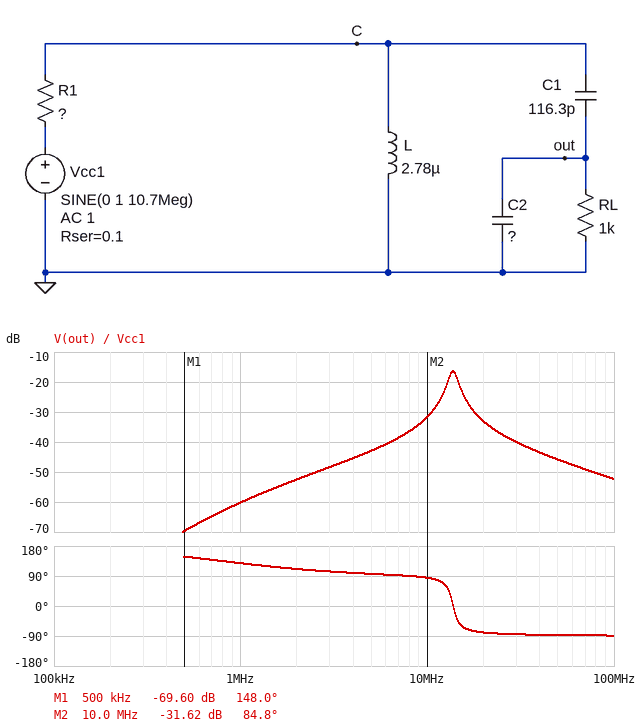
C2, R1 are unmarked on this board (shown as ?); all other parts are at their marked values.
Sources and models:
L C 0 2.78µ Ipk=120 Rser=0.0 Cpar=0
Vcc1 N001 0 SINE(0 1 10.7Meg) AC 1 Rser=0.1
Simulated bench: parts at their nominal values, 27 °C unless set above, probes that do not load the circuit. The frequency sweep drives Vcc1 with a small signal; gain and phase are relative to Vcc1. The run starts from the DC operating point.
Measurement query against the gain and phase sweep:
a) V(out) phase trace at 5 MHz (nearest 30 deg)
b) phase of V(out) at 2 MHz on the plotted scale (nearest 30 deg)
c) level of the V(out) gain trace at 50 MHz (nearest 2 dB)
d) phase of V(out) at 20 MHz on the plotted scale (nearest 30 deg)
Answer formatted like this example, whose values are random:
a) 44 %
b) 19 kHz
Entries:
a) 90 deg
b) 120 deg
c) -46 dB
d) -90 deg
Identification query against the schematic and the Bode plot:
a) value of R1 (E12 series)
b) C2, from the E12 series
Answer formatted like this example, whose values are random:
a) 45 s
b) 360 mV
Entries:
a) 8.2 kΩ
b) 82 pF
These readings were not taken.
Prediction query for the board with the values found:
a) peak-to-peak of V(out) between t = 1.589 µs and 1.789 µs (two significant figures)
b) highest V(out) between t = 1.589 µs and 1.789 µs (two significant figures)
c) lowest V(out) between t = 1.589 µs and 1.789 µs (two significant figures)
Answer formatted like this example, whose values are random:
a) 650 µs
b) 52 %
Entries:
a) 67 mV
b) 33 mV
c) -33 mV
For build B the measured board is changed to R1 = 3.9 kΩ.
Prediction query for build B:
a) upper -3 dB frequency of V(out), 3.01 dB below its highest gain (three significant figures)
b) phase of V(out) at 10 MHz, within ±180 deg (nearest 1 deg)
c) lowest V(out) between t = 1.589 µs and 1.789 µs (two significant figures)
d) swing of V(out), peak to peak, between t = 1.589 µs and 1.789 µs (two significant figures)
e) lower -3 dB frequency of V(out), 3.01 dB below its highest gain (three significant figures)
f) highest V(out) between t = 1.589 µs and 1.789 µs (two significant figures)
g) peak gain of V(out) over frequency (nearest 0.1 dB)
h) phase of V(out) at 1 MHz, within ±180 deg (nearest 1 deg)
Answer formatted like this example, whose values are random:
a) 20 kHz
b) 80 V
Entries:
a) 14.8 MHz
b) 82 deg
c) -69 mV
d) 140 mV
e) 12.8 MHz
f) 69 mV
g) -12.0 dB
h) 128 deg
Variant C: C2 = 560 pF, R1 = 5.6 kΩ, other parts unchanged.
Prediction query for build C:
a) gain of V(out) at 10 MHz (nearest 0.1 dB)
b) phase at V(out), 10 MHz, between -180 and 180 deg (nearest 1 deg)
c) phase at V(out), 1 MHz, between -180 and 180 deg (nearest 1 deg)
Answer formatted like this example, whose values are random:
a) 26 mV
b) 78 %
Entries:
a) -22.0 dB
b) -56 deg
c) 103 deg
